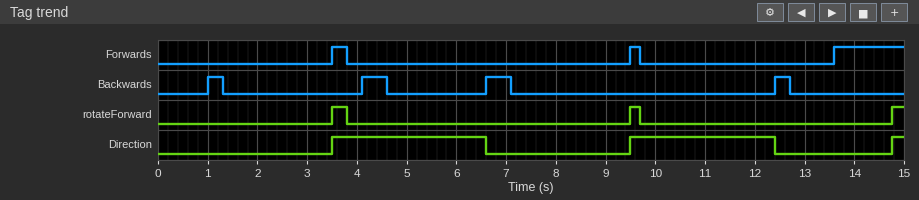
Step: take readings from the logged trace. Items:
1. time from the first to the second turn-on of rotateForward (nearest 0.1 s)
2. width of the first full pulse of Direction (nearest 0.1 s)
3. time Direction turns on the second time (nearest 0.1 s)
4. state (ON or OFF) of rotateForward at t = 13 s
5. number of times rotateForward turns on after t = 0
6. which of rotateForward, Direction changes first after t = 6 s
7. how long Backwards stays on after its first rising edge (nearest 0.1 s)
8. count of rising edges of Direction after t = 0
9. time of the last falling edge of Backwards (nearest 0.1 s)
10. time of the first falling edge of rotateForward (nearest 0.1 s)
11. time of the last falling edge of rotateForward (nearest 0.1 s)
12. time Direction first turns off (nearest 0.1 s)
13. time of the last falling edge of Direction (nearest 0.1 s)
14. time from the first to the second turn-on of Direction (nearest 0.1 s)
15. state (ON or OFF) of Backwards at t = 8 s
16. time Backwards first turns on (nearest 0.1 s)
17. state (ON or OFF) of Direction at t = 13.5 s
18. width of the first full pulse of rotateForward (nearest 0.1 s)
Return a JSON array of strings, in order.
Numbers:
["6.0 s", "3.1 s", "9.5 s", "OFF", "3", "Direction", "0.3 s", "3", "12.7 s", "3.8 s", "9.7 s", "6.6 s", "12.4 s", "6.0 s", "OFF", "1.0 s", "OFF", "0.3 s"]
